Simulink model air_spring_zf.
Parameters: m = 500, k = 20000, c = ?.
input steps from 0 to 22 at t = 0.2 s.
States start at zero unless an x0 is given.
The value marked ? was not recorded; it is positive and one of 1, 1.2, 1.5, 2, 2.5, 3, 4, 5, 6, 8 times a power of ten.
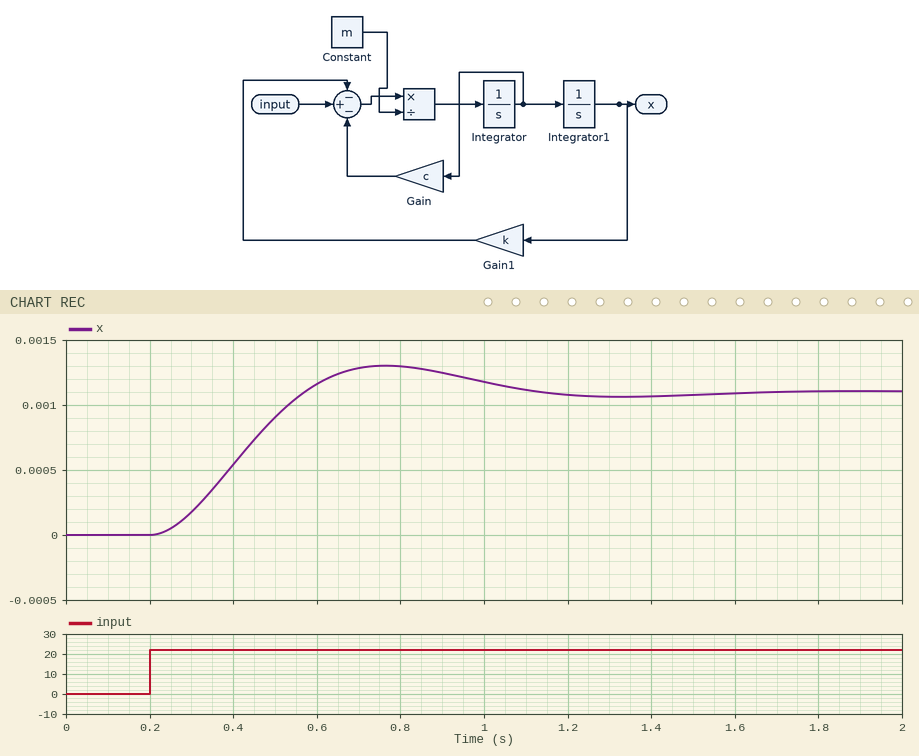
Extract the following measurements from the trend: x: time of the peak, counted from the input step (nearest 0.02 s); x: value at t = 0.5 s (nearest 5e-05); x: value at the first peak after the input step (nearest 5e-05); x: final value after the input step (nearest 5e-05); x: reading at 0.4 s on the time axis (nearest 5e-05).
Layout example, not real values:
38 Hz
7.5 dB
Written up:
0.56 s
0.00090
0.00130
0.00110
0.00055
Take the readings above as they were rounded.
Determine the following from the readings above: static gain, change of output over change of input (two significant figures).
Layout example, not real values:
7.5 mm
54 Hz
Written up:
0.000050
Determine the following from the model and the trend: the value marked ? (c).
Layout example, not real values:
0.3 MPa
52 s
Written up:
3000
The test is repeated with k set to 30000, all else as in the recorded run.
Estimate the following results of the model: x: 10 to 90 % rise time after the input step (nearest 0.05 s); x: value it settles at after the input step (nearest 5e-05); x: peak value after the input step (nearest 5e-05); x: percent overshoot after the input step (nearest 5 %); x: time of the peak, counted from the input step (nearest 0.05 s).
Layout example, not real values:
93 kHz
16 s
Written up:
0.20 s
0.00075
0.00095
25 %
0.45 s
